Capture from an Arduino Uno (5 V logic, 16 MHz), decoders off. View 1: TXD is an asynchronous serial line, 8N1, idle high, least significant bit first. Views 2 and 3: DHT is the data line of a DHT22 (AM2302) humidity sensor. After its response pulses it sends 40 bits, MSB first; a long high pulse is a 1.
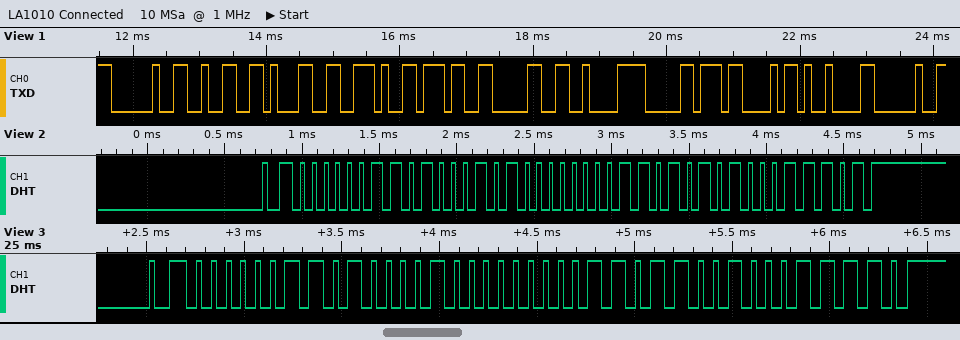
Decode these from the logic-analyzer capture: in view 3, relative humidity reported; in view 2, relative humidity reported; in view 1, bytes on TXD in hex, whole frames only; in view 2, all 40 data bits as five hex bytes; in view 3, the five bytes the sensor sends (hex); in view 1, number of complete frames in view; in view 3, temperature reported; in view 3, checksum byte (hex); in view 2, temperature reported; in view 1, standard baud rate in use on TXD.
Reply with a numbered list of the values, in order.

1. 83.4 %
2. 83.7 %
3. 20 32 31 2E 37 30 C2 B0 43 09 20
4. 03 45 00 D5 1D
5. 03 42 00 D9 1E
6. 11
7. 21.7 °C
8. 0x1E
9. 21.3 °C
10. 9600 baud
